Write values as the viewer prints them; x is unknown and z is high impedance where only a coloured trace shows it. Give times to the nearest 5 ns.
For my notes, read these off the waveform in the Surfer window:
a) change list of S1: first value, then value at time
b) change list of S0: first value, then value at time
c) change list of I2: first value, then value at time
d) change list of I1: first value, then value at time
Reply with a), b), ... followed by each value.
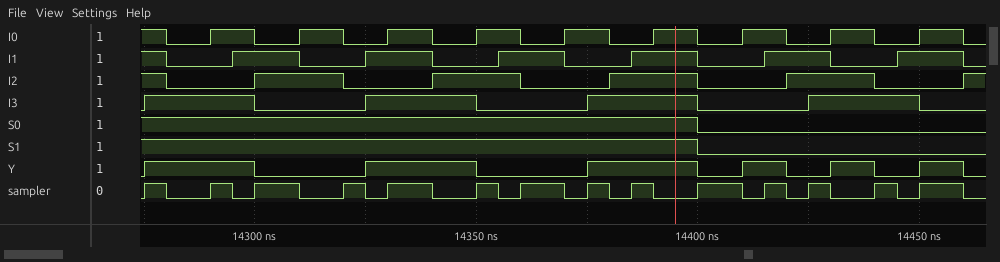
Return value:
a) 1, 0 at 14400 ns
b) 1, 0 at 14400 ns
c) 1, 0 at 14280 ns, 1 at 14300 ns, 0 at 14320 ns, 1 at 14340 ns, 0 at 14360 ns, 1 at 14380 ns, 0 at 14400 ns, 1 at 14420 ns, 0 at 14440 ns, 1 at 14460 ns
d) 1, 0 at 14280 ns, 1 at 14295 ns, 0 at 14310 ns, 1 at 14325 ns, 0 at 14340 ns, 1 at 14355 ns, 0 at 14370 ns, 1 at 14385 ns, 0 at 14400 ns, 1 at 14415 ns, 0 at 14430 ns, 1 at 14445 ns, 0 at 14460 ns
